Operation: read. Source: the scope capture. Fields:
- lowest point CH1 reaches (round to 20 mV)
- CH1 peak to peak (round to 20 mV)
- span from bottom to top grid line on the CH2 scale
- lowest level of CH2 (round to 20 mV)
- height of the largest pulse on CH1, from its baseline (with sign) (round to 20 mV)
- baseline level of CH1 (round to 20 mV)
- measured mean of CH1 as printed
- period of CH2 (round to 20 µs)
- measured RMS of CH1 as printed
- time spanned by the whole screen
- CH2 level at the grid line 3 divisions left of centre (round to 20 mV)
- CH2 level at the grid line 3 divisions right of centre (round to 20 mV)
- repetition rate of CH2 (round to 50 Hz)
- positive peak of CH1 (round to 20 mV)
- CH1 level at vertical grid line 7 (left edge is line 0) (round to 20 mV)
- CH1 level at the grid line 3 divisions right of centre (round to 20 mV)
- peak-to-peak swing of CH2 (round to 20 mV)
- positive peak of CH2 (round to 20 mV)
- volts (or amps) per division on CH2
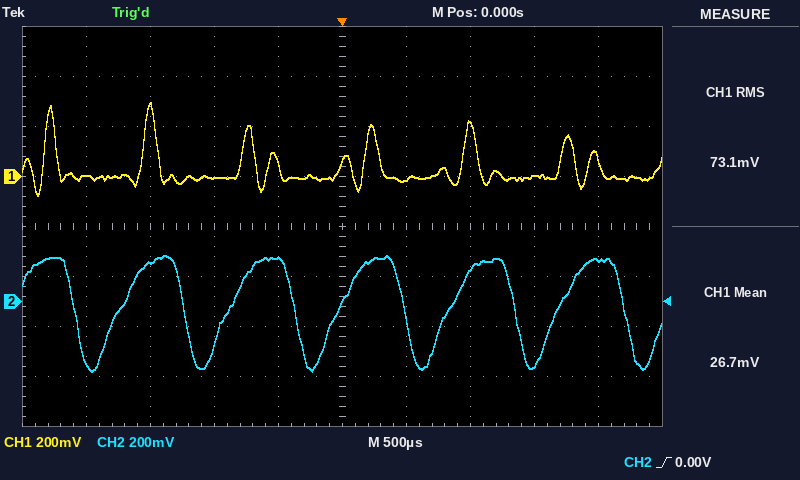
-80 mV
380 mV
1.6 V
-280 mV
+300 mV
0 mV
26.7 mV
860 µs
73.1 mV
5 ms
160 mV
-260 mV
1.15 kHz
300 mV
200 mV
0 mV
460 mV
180 mV
200 mV
